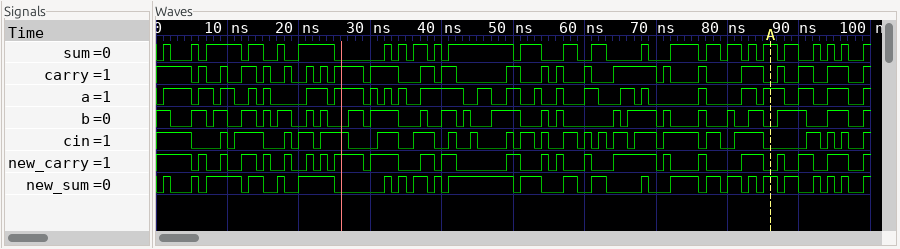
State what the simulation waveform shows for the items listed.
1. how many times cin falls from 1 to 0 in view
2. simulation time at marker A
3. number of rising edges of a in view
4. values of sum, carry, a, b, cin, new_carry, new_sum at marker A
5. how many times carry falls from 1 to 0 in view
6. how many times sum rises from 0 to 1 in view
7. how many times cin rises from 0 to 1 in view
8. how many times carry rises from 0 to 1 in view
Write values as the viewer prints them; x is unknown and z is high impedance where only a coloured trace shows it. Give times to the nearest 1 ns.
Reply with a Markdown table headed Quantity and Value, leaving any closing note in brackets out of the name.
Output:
| Quantity | Value |
|---|---|
| how many times cin falls from 1 to 0 in view | 24 |
| simulation time at marker A | 86 ns |
| number of rising edges of a in view | 24 |
| values of sum, carry, a, b, cin, new_carry, new_sum at marker A | sum=1, carry=0, a=1, b=0, cin=0, new_carry=0, new_sum=1 |
| how many times carry falls from 1 to 0 in view | 23 |
| how many times sum rises from 0 to 1 in view | 25 |
| how many times cin rises from 0 to 1 in view | 24 |
| how many times carry rises from 0 to 1 in view | 23 |
